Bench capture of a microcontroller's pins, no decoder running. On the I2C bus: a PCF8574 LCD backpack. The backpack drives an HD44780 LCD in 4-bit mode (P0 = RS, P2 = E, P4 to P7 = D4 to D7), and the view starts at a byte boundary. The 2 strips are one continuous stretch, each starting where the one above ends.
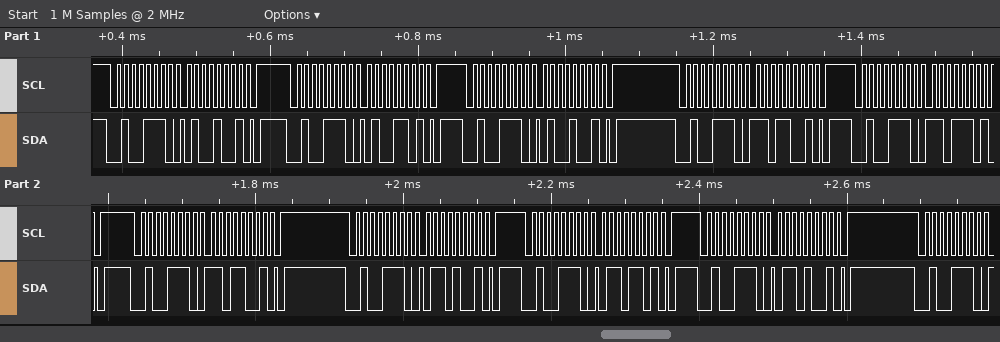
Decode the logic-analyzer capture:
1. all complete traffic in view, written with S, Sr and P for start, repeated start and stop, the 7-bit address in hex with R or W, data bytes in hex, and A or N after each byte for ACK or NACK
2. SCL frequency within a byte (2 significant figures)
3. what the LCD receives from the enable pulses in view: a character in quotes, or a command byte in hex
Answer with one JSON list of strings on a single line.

["S 27W A 49 A P S 27W A 4D A P S 27W A 49 A P S 27W A D9 A P S 27W A DD A P S 27W A D9 A P S 27W A 69 A P S 27W A 6D A P S 27W A 69 A P S 27W A", "100 kHz", "'M'"]
